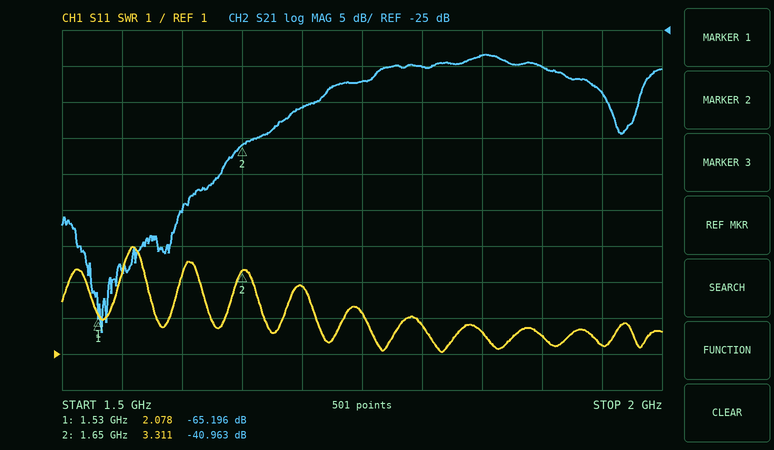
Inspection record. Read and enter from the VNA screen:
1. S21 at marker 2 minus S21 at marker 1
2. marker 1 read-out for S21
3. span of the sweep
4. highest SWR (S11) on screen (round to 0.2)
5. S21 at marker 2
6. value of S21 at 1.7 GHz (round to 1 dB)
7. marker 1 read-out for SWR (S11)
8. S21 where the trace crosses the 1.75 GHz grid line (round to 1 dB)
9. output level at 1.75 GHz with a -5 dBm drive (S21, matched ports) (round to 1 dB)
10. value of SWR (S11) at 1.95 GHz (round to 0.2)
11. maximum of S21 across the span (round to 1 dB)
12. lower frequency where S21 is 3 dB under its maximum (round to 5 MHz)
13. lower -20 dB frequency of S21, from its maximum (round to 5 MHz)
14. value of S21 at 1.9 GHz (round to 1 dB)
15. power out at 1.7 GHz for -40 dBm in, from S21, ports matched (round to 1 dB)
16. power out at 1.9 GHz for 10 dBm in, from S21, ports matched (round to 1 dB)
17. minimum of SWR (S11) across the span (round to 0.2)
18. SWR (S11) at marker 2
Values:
24.233 dB
-65.196 dB
500 MHz
4.0
-40.963 dB
-36 dB
2.078
-32 dB
-37 dBm
1.2
-28 dB
1.760 GHz
1.605 GHz
-30 dB
-76 dBm
-20 dBm
1.0
3.311
